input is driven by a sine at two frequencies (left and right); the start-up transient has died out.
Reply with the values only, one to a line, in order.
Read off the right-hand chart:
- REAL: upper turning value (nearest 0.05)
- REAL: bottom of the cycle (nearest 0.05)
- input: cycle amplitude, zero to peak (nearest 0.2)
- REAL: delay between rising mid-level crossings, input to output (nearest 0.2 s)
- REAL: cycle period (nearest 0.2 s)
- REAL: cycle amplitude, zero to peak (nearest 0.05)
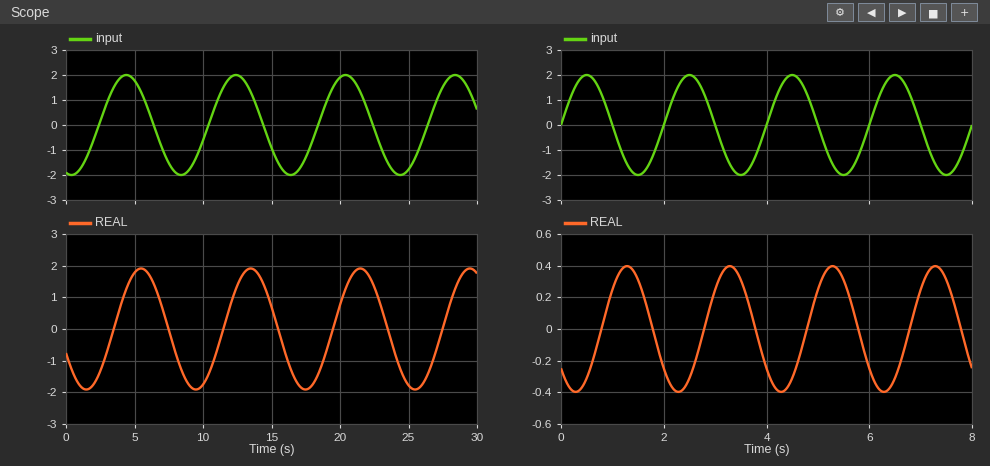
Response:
0.40
-0.40
2.0
0.8 s
2.0 s
0.40
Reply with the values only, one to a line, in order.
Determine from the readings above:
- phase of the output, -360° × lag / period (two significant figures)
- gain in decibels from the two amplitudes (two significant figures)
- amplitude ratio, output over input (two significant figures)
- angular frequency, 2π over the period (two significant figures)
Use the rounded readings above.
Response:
-140°
-14 dB
0.20
3.1 rad/s
